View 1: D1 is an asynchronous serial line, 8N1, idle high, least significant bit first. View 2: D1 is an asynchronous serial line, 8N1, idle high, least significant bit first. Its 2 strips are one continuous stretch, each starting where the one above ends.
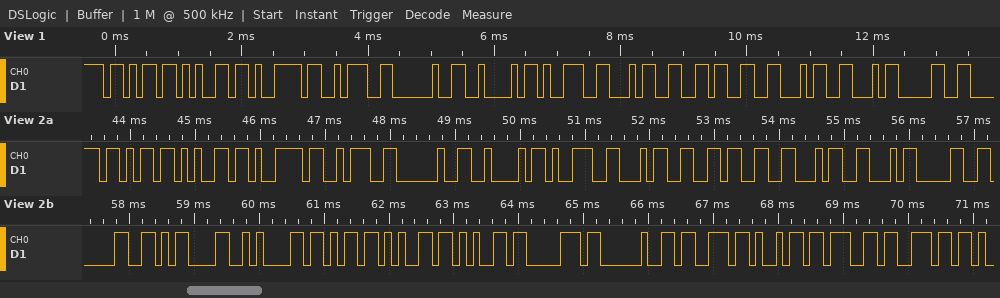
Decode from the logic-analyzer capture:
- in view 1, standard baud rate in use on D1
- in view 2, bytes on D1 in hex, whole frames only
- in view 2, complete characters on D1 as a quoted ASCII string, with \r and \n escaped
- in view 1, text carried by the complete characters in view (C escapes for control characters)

9600 baud
6B 65 79 3A 20 42 39 34 36 46 46 30 30 0D 0A 6B 65 65 70 20 73 69 67 6E
"key: B946FF00\r\nkeep sign"
"key: B946FF0"
